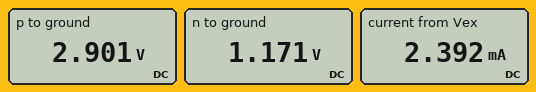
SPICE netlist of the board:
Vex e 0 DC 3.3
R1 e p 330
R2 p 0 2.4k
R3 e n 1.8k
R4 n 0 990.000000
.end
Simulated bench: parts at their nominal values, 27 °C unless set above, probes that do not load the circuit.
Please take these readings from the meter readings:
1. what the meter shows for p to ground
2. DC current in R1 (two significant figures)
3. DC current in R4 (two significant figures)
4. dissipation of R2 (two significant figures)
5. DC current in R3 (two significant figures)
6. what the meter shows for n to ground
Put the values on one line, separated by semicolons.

2.901 V; 1.2 mA; 1.2 mA; 3.5 mW; 1.2 mA; 1.171 V
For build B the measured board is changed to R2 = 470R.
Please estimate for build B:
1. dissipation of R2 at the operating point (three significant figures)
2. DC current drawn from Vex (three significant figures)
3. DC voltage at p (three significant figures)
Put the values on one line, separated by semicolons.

8.00 mW; 5.31 mA; 1.94 V
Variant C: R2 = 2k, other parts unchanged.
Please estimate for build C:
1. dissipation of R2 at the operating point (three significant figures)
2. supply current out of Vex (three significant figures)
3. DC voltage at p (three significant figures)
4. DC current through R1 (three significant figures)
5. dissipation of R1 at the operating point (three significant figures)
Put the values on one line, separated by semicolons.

4.01 mW; 2.60 mA; 2.83 V; 1.42 mA; 662 µW
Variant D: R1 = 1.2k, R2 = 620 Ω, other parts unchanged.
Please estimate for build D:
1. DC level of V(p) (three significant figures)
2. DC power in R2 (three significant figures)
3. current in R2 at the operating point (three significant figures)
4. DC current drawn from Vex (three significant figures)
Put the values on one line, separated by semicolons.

1.12 V; 2.04 mW; 1.81 mA; 3.00 mA
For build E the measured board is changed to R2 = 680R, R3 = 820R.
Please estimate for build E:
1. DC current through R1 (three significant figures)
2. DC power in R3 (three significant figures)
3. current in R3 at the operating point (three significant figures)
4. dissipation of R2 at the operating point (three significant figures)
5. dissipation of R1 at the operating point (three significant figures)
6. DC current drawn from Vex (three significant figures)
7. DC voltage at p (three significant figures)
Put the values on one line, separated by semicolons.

3.27 mA; 2.73 mW; 1.82 mA; 7.26 mW; 3.52 mW; 5.09 mA; 2.22 V
